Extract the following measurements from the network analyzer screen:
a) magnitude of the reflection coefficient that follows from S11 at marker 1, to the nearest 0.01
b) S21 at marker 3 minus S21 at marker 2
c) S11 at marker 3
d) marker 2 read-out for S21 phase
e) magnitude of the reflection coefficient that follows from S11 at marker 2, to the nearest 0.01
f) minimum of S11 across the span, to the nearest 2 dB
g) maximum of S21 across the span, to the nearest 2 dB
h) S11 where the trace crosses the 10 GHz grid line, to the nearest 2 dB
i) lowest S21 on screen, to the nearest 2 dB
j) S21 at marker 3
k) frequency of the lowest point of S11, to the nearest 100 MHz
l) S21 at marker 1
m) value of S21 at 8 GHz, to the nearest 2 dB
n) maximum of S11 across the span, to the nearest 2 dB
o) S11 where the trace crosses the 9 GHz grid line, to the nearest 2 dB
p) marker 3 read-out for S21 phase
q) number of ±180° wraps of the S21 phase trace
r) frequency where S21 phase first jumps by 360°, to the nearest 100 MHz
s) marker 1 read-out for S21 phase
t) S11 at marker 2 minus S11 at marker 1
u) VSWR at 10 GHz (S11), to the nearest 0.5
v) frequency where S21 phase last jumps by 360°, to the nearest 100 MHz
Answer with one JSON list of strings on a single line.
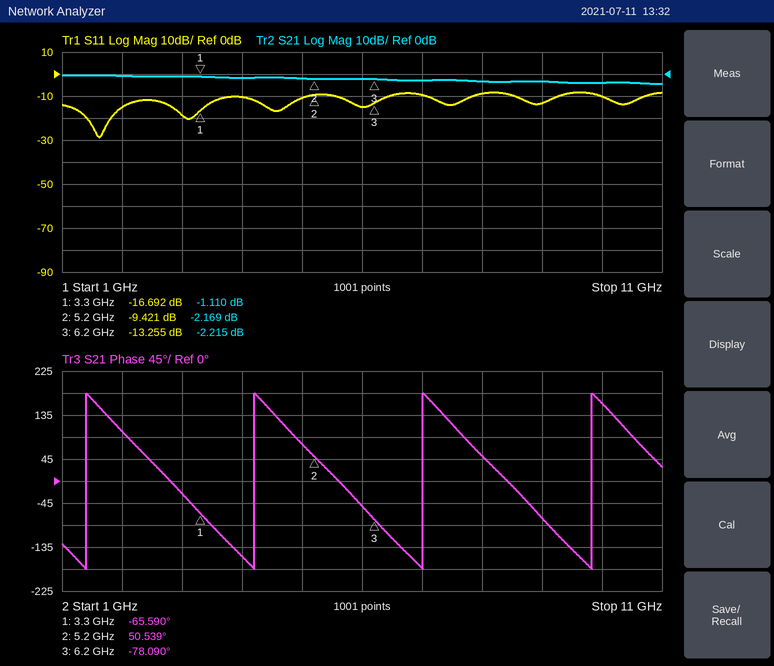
["0.15", "-0.046 dB", "-13.255 dB", "50.539°", "0.34", "-28 dB", "0 dB", "-10 dB", "-4 dB", "-2.215 dB", "1.6 GHz", "-1.110 dB", "-4 dB", "-8 dB", "-14 dB", "-78.090°", "4", "1.4 GHz", "-65.590°", "7.271 dB", "2.0", "9.8 GHz"]
